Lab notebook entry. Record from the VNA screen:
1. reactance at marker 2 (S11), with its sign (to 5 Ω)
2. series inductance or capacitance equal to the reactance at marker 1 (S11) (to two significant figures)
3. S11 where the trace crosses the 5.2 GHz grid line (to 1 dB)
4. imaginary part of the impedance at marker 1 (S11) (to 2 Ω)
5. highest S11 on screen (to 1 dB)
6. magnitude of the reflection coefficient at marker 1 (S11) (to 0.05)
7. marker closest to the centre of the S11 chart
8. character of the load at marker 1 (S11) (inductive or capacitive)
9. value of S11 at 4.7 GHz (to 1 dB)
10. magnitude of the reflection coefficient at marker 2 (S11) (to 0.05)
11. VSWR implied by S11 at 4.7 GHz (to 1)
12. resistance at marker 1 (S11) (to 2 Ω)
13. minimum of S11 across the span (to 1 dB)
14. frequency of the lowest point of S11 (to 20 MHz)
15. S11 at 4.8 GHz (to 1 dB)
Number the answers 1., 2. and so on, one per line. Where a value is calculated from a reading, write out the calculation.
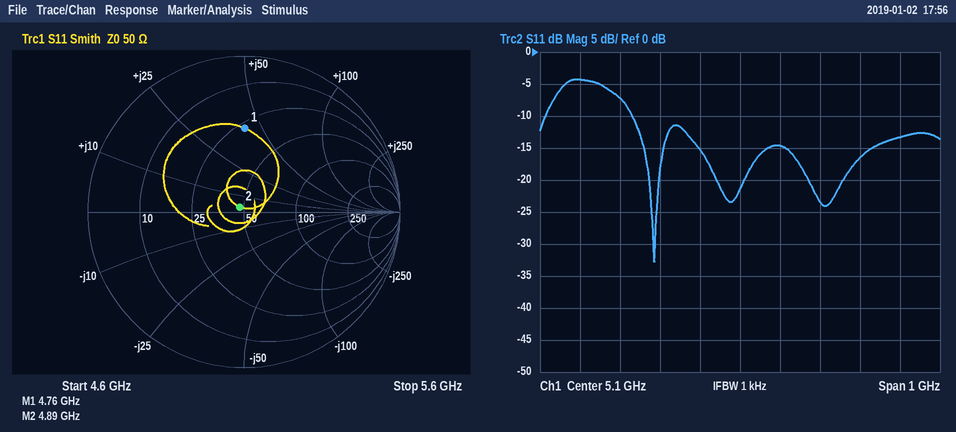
1. +5 Ω
2. L = 42 Ω/(2π × 4.76 GHz) ≈ 1.4 nH
3. -15 dB
4. +42 Ω
5. -4 dB
6. 0.55
7. marker 2
8. inductive
9. -4 dB
10. 0.05
11. |Γ| = 10^(-4/20) = 0.6310; VSWR = (1 + 0.6310)/(1 − 0.6310) ≈ 4
12. 28 Ω
13. -33 dB
14. 4.88 GHz
15. -7 dB
